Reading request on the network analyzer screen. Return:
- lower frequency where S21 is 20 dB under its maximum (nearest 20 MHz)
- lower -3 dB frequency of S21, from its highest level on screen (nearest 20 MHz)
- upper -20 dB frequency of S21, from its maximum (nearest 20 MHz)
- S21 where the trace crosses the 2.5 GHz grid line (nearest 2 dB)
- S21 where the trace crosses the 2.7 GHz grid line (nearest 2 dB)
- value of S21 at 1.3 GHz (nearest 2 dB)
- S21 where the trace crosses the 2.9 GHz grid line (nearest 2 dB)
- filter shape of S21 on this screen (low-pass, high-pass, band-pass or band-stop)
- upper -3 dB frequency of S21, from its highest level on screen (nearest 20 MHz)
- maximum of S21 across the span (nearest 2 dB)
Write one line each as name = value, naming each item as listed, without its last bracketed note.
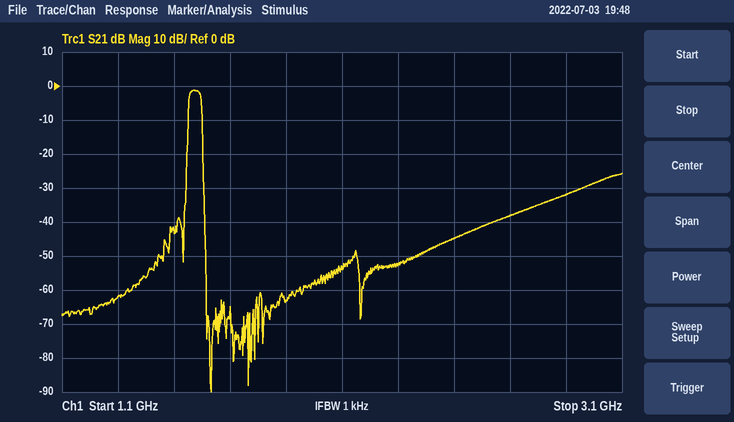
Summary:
lower frequency where S21 is 20 dB under its maximum = 1.54 GHz
lower -3 dB frequency of S21, from its highest level on screen = 1.56 GHz
upper -20 dB frequency of S21, from its maximum = 1.60 GHz
S21 where the trace crosses the 2.5 GHz grid line = -44 dB
S21 where the trace crosses the 2.7 GHz grid line = -38 dB
value of S21 at 1.3 GHz = -62 dB
S21 where the trace crosses the 2.9 GHz grid line = -32 dB
filter shape of S21 on this screen = band-pass
upper -3 dB frequency of S21, from its highest level on screen = 1.60 GHz
maximum of S21 across the span = -2 dB
